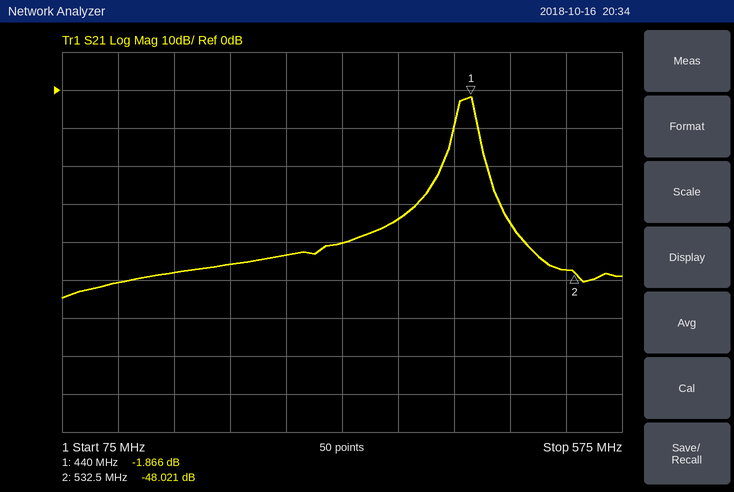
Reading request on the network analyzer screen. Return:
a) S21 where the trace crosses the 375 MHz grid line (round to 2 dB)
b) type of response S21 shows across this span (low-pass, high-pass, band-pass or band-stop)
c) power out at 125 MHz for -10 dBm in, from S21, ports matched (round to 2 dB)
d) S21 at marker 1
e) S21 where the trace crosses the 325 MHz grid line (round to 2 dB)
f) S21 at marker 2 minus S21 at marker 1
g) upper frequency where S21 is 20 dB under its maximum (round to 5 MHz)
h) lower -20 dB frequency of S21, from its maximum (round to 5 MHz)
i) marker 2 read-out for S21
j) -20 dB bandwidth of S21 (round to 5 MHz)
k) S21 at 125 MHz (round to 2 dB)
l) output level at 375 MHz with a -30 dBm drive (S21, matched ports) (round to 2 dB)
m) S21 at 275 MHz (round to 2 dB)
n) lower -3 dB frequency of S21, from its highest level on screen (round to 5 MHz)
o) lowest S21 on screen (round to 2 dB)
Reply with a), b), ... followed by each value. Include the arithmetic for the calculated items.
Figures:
a) -34 dB
b) band-pass
c) -10 dBm + (-50 dB) = -60 dBm
d) -1.866 dB
e) -40 dB
f) -48.021 − (-1.866) = -46.155 dB
g) 455 MHz
h) 410 MHz
i) -48.021 dB
j) 455 MHz − 410 MHz = 45 MHz
k) -50 dB
l) -30 dBm + (-34 dB) = -64 dBm
m) -44 dB
n) 430 MHz
o) -54 dB
